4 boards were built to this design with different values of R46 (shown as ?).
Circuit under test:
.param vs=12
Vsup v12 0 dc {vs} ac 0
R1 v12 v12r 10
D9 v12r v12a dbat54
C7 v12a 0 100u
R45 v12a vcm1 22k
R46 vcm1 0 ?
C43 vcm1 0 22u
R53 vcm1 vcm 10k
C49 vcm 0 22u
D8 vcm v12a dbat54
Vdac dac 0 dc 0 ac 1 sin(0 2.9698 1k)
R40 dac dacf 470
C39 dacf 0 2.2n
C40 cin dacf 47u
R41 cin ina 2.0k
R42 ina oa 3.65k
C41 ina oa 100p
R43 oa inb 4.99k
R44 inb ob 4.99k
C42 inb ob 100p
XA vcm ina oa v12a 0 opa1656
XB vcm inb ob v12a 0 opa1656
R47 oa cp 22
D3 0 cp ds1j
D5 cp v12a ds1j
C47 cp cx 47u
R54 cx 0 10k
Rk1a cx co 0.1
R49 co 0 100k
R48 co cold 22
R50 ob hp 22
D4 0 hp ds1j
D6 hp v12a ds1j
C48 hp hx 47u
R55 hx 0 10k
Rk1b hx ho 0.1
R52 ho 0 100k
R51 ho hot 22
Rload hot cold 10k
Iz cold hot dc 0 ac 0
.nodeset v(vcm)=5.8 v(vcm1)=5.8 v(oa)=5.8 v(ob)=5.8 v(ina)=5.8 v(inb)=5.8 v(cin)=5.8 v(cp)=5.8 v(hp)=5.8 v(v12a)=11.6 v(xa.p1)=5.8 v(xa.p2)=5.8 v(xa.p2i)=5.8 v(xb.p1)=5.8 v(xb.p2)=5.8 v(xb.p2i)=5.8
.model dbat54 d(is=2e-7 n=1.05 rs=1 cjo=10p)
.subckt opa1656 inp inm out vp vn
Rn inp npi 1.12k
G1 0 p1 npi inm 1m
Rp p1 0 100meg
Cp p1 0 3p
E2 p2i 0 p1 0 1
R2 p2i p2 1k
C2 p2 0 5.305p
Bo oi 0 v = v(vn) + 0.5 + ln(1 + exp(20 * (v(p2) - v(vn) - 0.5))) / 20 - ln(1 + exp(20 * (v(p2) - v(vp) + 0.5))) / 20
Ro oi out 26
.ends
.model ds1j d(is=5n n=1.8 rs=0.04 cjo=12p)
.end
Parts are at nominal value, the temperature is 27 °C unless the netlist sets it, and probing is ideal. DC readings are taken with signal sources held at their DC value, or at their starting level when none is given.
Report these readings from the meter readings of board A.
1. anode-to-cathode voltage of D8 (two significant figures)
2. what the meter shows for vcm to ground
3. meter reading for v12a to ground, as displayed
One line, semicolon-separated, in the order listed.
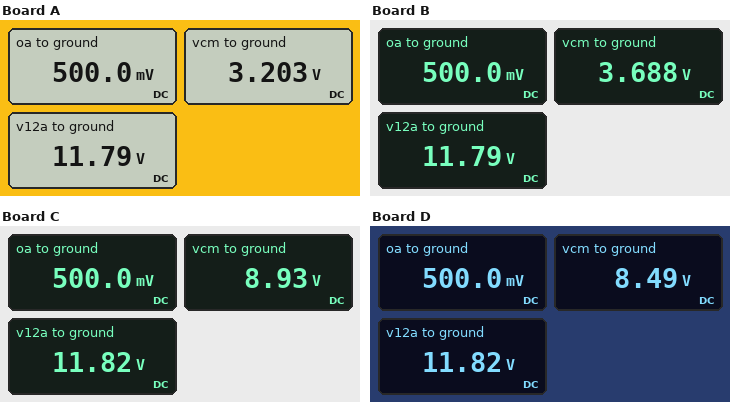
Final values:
-8.6 V; 3.203 V; 11.79 V
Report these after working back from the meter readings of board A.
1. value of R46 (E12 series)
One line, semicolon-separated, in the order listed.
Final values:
8.2 kΩ
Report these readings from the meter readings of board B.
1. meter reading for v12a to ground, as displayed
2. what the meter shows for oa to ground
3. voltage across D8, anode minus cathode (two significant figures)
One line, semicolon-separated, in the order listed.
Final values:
11.79 V; 500.0 mV; -8.1 V
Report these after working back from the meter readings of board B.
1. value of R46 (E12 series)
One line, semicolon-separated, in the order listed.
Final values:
10 kΩ
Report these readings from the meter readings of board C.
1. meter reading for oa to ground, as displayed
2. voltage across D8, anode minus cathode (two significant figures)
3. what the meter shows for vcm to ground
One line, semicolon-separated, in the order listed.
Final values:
500.0 mV; -2.9 V; 8.93 V
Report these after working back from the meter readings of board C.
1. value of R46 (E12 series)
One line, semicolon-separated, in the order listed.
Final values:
68 kΩ
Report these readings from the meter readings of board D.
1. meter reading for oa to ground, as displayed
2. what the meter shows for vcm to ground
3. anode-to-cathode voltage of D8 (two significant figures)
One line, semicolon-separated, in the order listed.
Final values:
500.0 mV; 8.49 V; -3.3 V
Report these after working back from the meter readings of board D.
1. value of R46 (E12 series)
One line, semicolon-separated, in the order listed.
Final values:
56 kΩ
